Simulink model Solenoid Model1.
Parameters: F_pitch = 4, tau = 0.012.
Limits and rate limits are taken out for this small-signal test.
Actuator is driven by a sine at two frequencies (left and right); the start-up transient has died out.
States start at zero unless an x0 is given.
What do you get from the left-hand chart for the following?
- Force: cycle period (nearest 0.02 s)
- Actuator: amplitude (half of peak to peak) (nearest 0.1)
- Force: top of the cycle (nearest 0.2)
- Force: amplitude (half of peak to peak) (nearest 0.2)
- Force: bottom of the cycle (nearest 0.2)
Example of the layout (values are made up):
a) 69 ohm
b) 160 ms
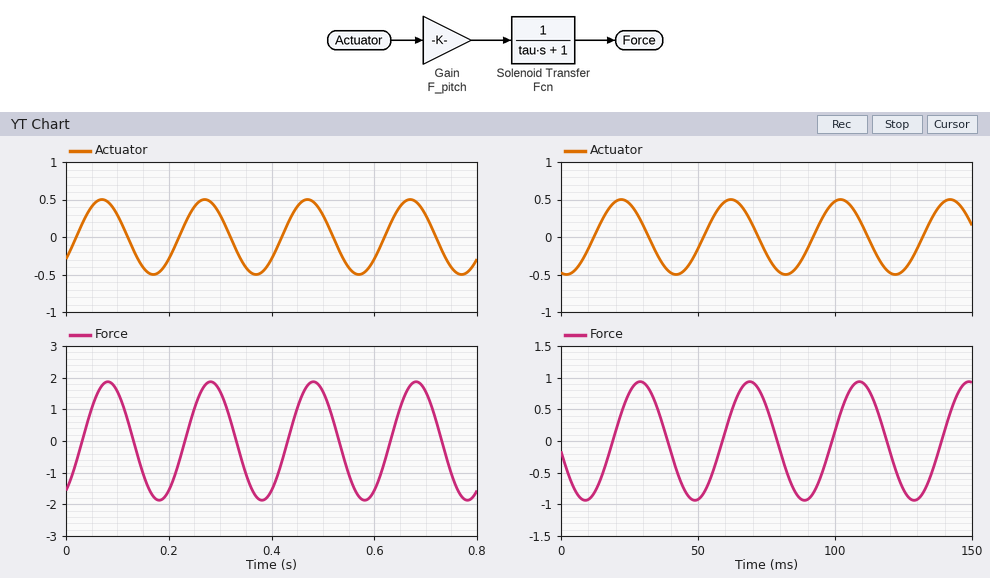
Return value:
a) 0.20 s
b) 0.5
c) 1.8
d) 1.8
e) -1.8
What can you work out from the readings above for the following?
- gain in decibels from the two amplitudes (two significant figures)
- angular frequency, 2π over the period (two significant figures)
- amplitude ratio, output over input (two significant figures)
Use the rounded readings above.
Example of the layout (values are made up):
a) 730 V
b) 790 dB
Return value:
a) 11 dB
b) 31 rad/s
c) 3.6
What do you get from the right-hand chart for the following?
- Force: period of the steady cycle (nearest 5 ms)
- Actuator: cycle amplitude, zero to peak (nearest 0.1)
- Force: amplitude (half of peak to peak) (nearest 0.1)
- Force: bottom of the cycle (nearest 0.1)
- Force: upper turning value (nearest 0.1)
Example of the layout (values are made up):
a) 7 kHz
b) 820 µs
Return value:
a) 40 ms
b) 0.5
c) 0.9
d) -0.9
e) 0.9
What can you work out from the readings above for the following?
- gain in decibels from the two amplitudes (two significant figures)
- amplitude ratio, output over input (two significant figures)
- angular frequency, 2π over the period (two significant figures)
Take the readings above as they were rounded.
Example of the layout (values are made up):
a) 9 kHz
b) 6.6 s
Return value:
a) 5.1 dB
b) 1.8
c) 0.16 rad/ms
